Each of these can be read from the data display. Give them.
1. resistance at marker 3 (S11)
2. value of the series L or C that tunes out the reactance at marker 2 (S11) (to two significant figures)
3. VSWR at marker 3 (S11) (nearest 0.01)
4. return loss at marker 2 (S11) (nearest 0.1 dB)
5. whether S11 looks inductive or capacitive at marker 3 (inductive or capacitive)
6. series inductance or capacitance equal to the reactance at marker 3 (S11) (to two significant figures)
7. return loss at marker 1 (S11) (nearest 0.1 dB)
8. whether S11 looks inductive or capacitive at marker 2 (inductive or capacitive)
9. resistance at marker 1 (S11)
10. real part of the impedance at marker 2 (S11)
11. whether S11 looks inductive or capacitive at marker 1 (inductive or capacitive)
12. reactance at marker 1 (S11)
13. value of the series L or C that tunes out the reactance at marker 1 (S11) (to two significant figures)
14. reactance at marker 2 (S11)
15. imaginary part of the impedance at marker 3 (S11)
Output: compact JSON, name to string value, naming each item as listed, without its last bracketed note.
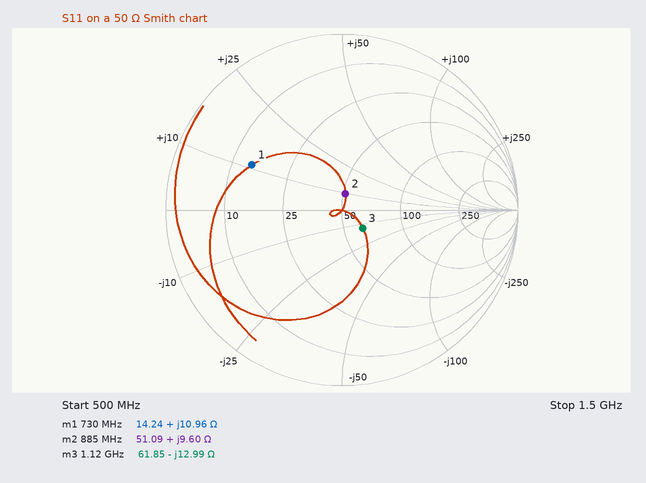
{"resistance at marker 3": "61.85 Ω", "value of the series L or C that tunes out the reactance at marker 2 (S11)": "19 pF", "VSWR at marker 3 (S11)": "1.37", "return loss at marker 2 (S11)": "20.4 dB", "whether S11 looks inductive or capacitive at marker 3": "capacitive", "series inductance or capacitance equal to the reactance at marker 3 (S11)": "11 pF", "return loss at marker 1 (S11)": "4.8 dB", "whether S11 looks inductive or capacitive at marker 2": "inductive", "resistance at marker 1": "14.24 Ω", "real part of the impedance at marker 2": "51.09 Ω", "whether S11 looks inductive or capacitive at marker 1": "inductive", "reactance at marker 1": "+10.96 Ω", "value of the series L or C that tunes out the reactance at marker 1 (S11)": "20 pF", "reactance at marker 2": "+9.60 Ω", "imaginary part of the impedance at marker 3": "-12.99 Ω"}
